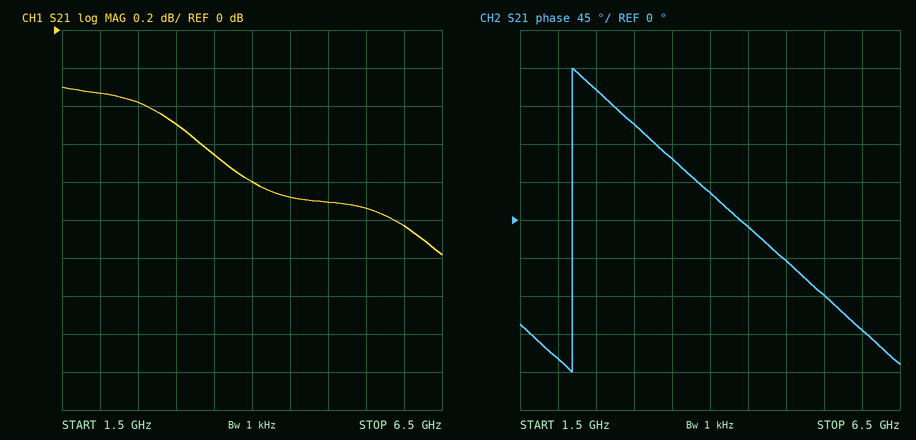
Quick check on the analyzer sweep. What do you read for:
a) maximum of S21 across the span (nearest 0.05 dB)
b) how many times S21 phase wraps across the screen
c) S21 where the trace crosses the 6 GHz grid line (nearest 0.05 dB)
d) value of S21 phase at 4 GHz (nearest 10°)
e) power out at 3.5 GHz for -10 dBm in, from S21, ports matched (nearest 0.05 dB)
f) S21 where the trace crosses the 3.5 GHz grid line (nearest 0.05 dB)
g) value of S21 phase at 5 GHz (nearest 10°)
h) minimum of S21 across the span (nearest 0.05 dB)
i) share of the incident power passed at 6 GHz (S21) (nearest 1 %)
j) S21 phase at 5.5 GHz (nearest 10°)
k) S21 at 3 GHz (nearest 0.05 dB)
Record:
-0.30 dB
1
-1.05 dB
30°
-10.65 dBm
-0.65 dB
-50°
-1.20 dB
79 %
-90°
-0.50 dB
